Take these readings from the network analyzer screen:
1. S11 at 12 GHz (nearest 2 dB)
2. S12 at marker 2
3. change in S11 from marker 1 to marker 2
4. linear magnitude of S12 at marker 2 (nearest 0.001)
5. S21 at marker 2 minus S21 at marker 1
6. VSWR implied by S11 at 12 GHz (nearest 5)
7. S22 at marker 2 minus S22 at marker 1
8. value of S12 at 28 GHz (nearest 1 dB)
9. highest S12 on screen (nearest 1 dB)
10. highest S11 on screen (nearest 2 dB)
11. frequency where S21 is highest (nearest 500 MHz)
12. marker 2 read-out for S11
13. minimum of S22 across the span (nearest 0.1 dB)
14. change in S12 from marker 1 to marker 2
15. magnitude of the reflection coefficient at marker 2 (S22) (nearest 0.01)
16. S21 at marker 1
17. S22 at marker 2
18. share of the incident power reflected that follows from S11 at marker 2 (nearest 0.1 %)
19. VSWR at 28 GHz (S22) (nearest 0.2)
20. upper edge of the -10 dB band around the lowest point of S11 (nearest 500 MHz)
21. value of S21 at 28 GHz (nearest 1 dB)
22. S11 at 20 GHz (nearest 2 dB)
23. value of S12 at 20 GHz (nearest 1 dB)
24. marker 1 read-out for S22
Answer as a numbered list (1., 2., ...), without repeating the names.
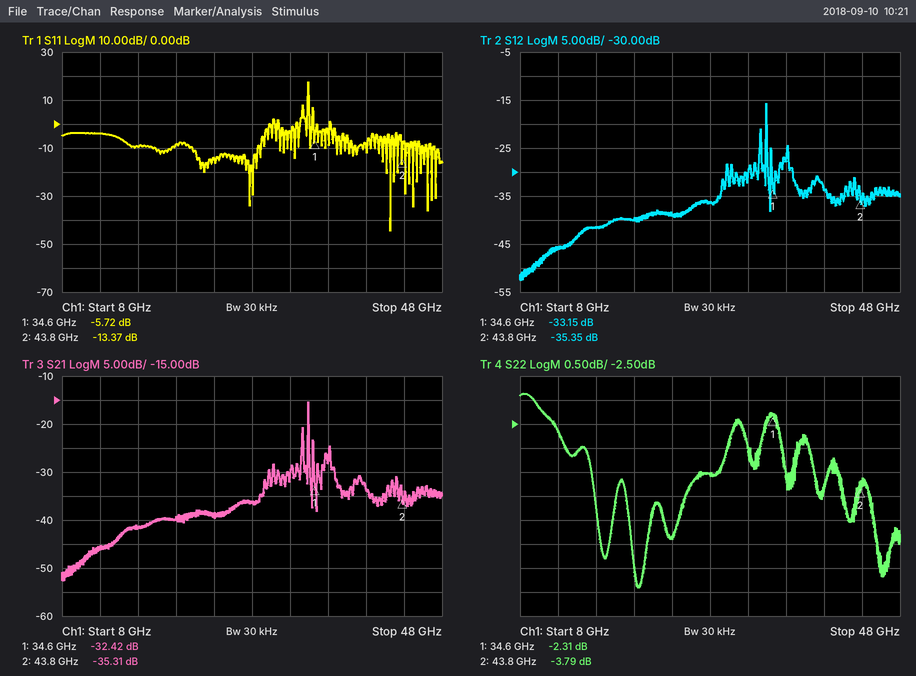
1. -4 dB
2. -35.35 dB
3. -7.65 dB
4. 0.017
5. -2.89 dB
6. 5
7. -1.48 dB
8. -36 dB
9. -16 dB
10. 18 dB
11. 34.0 GHz
12. -13.37 dB
13. -5.9 dB
14. -2.20 dB
15. 0.65
16. -32.42 dB
17. -3.79 dB
18. 4.6 %
19. 5.0
20. 42.5 GHz
21. -36 dB
22. -8 dB
23. -40 dB
24. -2.31 dB
